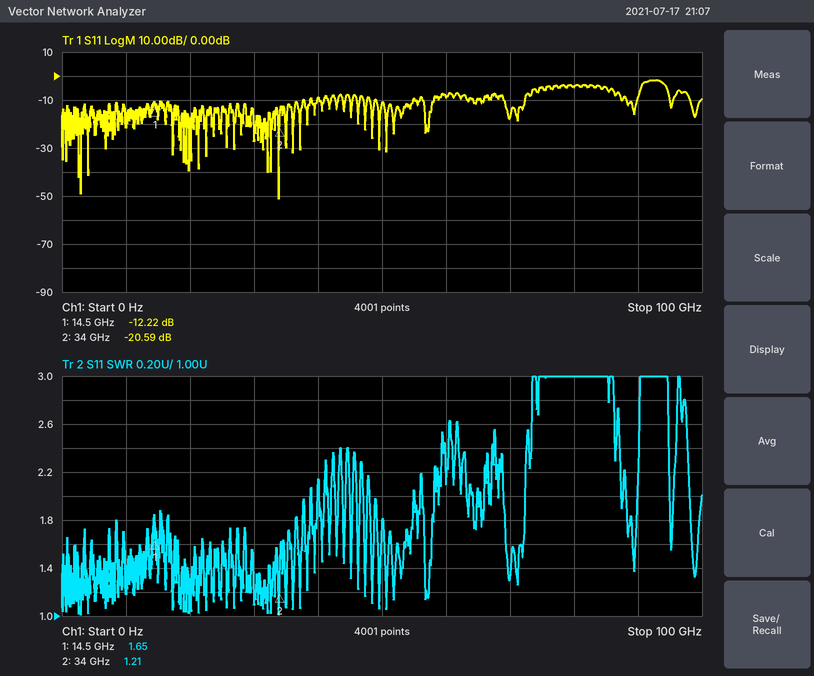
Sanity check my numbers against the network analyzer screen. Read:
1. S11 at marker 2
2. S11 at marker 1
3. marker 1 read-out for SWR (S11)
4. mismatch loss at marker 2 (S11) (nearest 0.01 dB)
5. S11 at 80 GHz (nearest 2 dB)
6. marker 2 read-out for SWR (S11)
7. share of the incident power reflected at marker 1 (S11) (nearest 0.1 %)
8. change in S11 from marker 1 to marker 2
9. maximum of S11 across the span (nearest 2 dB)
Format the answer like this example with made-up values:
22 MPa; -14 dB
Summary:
-20.59 dB; -12.22 dB; 1.65; 0.04 dB; -4 dB; 1.21; 6.0 %; -8.37 dB; -2 dB
